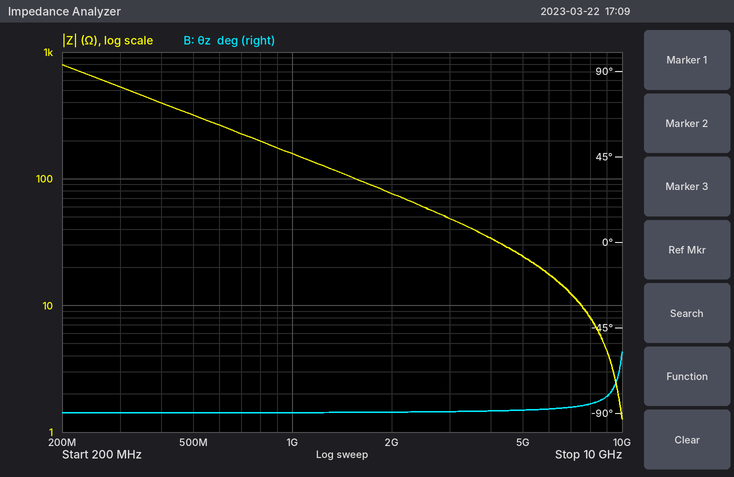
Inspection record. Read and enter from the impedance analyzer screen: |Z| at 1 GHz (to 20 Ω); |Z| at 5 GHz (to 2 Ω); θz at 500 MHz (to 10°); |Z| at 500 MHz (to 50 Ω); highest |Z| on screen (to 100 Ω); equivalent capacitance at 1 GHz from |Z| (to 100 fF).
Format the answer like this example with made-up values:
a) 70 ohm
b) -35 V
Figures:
a) 160 Ω
b) 24 Ω
c) -90°
d) 300 Ω
e) 800 Ω
f) 1.0 pF
